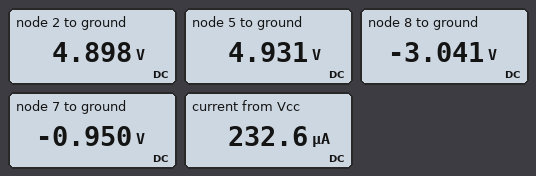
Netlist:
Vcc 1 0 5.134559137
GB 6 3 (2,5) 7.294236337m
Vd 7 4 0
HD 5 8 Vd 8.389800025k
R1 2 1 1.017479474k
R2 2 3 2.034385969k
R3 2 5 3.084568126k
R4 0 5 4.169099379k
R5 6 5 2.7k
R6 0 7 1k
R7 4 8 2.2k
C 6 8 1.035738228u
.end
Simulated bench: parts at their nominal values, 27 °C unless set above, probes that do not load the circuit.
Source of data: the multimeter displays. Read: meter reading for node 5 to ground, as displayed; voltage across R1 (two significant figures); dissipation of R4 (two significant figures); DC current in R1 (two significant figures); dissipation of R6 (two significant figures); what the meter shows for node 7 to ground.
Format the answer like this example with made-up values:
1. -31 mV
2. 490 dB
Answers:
1. 4.931 V
2. 240 mV
3. 5.8 mW
4. 230 µA
5. 900 µW
6. -0.950 V
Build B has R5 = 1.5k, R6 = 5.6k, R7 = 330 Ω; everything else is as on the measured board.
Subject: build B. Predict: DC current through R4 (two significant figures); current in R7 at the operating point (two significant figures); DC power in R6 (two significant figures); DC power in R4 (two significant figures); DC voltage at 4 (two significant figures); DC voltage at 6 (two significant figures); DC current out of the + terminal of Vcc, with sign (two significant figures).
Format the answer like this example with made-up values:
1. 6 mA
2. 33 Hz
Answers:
1. 1.4 mA
2. 2.4 mA
3. 33 mW
4. 8.7 mW
5. -14 V
6. 4.4 V
7. -1.0 mA
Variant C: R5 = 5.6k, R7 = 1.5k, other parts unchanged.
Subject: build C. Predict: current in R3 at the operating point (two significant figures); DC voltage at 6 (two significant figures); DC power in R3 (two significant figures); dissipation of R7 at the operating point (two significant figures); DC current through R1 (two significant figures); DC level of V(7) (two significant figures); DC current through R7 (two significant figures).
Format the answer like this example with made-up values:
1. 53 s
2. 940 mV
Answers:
1. 16 µA
2. 6.8 V
3. 770 nW
4. 1.0 mW
5. 340 µA
6. -820 mV
7. 820 µA
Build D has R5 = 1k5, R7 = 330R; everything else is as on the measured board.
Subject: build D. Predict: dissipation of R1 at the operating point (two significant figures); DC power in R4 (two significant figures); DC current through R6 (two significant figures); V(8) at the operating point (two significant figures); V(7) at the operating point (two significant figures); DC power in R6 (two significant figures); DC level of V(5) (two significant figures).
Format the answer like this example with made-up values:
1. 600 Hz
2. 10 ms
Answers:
1. 220 µW
2. 5.4 mW
3. 670 µA
4. -890 mV
5. -670 mV
6. 450 µW
7. 4.7 V
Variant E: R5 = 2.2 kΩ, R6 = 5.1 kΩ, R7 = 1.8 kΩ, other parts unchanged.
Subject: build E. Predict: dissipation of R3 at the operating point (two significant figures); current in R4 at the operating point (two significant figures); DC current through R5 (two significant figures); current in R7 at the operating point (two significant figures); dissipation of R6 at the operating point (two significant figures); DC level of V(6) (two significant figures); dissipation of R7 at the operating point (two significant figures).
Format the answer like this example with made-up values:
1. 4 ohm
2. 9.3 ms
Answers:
1. 84 µW
2. 2.0 mA
3. 3.7 mA
4. 5.5 mA
5. 160 mW
6. 56 mV
7. 55 mW
